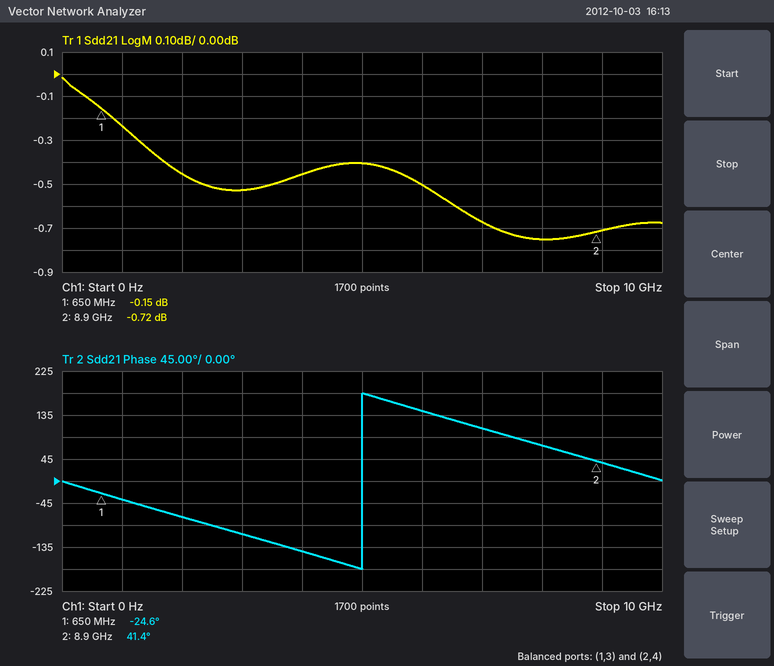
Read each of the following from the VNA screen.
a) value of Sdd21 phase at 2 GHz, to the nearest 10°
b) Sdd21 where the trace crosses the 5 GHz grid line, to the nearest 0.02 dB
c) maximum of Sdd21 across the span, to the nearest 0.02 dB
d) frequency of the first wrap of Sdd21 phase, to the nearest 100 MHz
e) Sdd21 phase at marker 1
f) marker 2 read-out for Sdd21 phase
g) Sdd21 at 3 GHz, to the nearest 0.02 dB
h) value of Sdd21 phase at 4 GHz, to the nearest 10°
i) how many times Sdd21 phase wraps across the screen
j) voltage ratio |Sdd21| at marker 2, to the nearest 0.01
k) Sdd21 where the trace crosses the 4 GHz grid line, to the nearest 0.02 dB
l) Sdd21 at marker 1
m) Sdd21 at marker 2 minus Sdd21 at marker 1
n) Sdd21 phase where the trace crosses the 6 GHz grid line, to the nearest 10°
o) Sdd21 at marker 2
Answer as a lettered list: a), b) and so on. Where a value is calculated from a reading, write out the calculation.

a) -70°
b) -0.40 dB
c) -0.02 dB
d) 5.0 GHz
e) -24.6°
f) 41.4°
g) -0.52 dB
h) -140°
i) 1
j) 10^(-0.72/20) ≈ 0.92
k) -0.46 dB
l) -0.15 dB
m) -0.72 − (-0.15) = -0.57 dB
n) 140°
o) -0.72 dB
